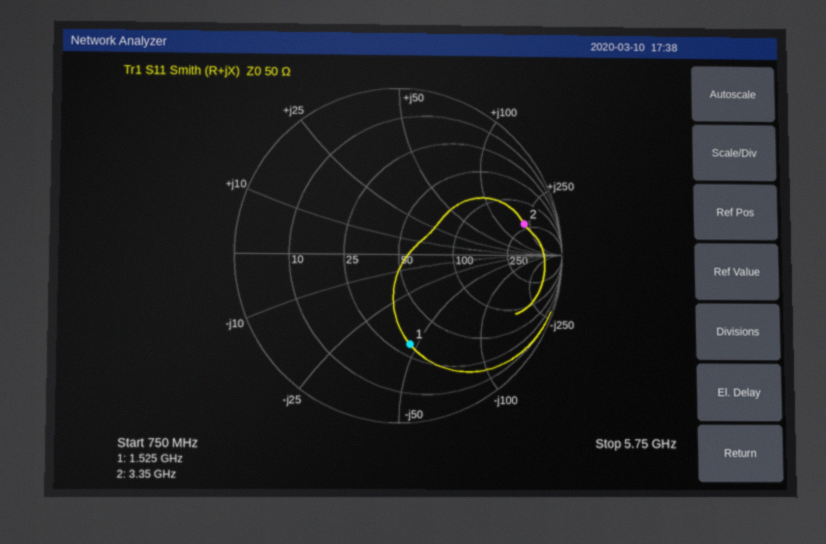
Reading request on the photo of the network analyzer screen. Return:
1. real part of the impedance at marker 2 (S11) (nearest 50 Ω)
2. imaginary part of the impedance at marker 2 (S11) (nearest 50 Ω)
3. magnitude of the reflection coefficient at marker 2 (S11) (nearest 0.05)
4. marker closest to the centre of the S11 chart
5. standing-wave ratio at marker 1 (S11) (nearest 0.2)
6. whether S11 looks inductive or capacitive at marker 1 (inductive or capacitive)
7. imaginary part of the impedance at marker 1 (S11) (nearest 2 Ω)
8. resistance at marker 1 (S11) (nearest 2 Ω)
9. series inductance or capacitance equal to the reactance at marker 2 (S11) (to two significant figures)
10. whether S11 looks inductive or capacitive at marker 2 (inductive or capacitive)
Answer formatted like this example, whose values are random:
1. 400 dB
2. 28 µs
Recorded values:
1. 200 Ω
2. +200 Ω
3. 0.80
4. marker 1
5. 3.4
6. capacitive
7. -46 Ω
8. 30 Ω
9. 10 nH
10. inductive
